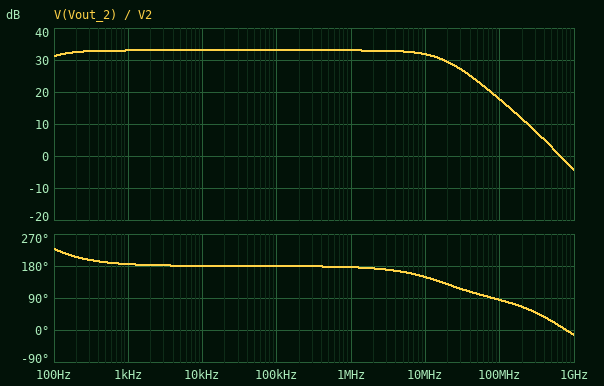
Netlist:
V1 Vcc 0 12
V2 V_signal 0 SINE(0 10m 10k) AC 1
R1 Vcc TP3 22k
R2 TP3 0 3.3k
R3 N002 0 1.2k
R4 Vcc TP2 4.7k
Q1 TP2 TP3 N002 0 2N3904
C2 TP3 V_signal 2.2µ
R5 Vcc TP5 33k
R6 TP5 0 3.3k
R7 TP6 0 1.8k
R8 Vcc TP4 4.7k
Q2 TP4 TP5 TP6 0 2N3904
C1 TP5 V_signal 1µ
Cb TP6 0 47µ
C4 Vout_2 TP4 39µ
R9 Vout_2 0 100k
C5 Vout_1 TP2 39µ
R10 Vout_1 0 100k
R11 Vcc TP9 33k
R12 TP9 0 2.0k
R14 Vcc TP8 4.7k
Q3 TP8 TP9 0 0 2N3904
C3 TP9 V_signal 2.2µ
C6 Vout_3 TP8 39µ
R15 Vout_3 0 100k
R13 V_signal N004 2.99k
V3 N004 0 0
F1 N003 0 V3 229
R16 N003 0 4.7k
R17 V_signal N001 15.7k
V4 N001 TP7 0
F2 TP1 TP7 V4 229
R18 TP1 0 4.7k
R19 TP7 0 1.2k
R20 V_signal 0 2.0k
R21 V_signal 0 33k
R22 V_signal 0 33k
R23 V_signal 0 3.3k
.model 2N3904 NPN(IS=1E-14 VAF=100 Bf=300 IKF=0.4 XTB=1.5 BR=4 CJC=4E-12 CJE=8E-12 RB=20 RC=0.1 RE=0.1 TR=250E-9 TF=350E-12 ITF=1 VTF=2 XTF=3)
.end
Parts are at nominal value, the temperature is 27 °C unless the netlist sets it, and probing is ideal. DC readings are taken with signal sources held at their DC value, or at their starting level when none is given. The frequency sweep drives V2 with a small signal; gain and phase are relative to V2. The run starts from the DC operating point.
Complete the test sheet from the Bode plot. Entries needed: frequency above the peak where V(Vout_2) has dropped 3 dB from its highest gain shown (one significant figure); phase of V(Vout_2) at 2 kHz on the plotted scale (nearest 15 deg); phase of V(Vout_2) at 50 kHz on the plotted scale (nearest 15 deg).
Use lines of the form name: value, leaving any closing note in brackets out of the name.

frequency above the peak where V(Vout_2) has dropped 3 dB from its highest gain shown: 20 MHz
phase of V(Vout_2) at 2 kHz on the plotted scale: 180 deg
phase of V(Vout_2) at 50 kHz on the plotted scale: 180 deg
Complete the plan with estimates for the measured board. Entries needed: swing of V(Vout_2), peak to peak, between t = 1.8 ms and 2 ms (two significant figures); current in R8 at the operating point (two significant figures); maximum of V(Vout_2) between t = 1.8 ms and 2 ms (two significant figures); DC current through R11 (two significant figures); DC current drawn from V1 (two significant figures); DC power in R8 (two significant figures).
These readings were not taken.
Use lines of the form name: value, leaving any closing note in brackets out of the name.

swing of V(Vout_2), peak to peak, between t = 1.8 ms and 2 ms: 900 mV
current in R8 at the operating point: 260 µA
maximum of V(Vout_2) between t = 1.8 ms and 2 ms: 380 mV
DC current through R11: 340 µA
DC current drawn from V1: 4.2 mA
DC power in R8: 320 µW
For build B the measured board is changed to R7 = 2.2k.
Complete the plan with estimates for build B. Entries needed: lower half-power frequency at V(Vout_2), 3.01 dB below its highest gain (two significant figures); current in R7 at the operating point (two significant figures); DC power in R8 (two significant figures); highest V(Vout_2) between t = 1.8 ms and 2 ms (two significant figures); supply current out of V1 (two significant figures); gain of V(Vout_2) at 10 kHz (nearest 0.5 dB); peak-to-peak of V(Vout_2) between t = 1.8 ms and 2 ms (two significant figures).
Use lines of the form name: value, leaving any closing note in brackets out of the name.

lower half-power frequency at V(Vout_2), 3.01 dB below its highest gain: 70 Hz
current in R7 at the operating point: 220 µA
DC power in R8: 220 µW
highest V(Vout_2) between t = 1.8 ms and 2 ms: 320 mV
supply current out of V1: 4.1 mA
gain of V(Vout_2) at 10 kHz: 31.5 dB
peak-to-peak of V(Vout_2) between t = 1.8 ms and 2 ms: 750 mV
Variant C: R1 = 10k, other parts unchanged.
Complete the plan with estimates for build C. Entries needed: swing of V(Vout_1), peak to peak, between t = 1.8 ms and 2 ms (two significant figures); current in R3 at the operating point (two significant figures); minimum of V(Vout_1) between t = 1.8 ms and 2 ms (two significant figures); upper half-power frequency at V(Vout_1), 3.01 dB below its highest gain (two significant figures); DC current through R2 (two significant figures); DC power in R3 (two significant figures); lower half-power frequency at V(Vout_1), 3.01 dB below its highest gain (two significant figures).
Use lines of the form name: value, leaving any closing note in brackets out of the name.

swing of V(Vout_1), peak to peak, between t = 1.8 ms and 2 ms: 74 mV
current in R3 at the operating point: 1.9 mA
minimum of V(Vout_1) between t = 1.8 ms and 2 ms: -37 mV
upper half-power frequency at V(Vout_1), 3.01 dB below its highest gain: 9.9 MHz
DC current through R2: 900 µA
DC power in R3: 4.4 mW
lower half-power frequency at V(Vout_1), 3.01 dB below its highest gain: 29 Hz
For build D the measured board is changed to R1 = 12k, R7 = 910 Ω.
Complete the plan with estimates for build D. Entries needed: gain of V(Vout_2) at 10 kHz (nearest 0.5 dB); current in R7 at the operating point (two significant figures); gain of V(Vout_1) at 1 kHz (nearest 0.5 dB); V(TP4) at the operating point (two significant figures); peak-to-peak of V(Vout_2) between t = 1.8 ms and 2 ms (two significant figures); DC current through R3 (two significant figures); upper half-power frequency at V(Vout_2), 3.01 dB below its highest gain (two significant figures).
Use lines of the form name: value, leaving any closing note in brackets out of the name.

gain of V(Vout_2) at 10 kHz: 38.5 dB
current in R7 at the operating point: 500 µA
gain of V(Vout_1) at 1 kHz: 11.5 dB
V(TP4) at the operating point: 9.7 V
peak-to-peak of V(Vout_2) between t = 1.8 ms and 2 ms: 1.7 V
DC current through R3: 1.6 mA
upper half-power frequency at V(Vout_2), 3.01 dB below its highest gain: 15 MHz
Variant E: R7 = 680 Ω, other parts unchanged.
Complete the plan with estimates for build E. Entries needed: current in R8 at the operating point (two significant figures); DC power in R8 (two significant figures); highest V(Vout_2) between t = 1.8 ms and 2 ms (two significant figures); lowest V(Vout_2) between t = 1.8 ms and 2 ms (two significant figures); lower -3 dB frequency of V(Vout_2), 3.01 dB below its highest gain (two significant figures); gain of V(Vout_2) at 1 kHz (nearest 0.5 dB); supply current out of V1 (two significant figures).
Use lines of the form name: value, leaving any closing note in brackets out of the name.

current in R8 at the operating point: 650 µA
DC power in R8: 2.0 mW
highest V(Vout_2) between t = 1.8 ms and 2 ms: 960 mV
lowest V(Vout_2) between t = 1.8 ms and 2 ms: -1.2 V
lower -3 dB frequency of V(Vout_2), 3.01 dB below its highest gain: 120 Hz
gain of V(Vout_2) at 1 kHz: 40.5 dB
supply current out of V1: 4.6 mA
